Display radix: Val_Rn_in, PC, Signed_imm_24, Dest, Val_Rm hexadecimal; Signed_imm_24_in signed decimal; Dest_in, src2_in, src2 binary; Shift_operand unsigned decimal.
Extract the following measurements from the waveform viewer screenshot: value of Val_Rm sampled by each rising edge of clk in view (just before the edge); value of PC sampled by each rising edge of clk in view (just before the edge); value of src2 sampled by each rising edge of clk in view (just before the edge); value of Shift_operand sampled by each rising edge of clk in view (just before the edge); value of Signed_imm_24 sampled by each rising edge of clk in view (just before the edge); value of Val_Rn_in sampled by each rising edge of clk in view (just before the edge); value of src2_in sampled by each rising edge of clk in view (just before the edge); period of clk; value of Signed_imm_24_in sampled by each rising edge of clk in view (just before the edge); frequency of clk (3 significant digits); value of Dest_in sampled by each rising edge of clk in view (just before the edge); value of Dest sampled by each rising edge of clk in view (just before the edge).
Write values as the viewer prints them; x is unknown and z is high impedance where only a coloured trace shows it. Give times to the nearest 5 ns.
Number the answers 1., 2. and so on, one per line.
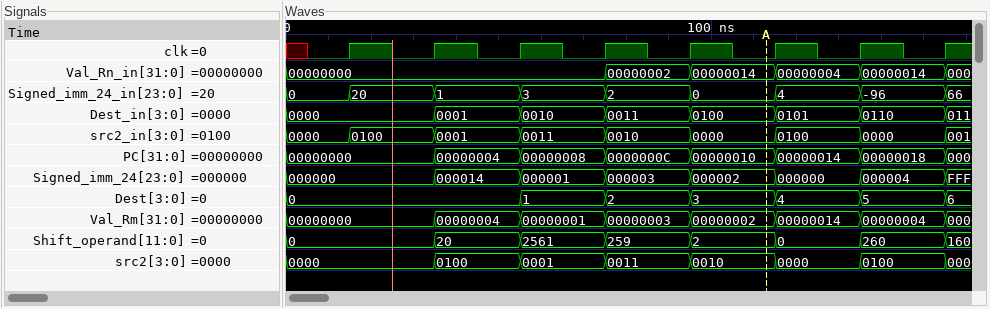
1. 00000000, 00000000, 00000004, 00000001, 00000003, 00000002, 00000014, 00000004
2. 00000000, 00000000, 00000004, 00000008, 0000000C, 00000010, 00000014, 00000018
3. 0000, 0000, 0100, 0001, 0011, 0010, 0000, 0100
4. 0, 0, 20, 2561, 259, 2, 0, 260
5. 000000, 000000, 000014, 000001, 000003, 000002, 000000, 000004
6. 00000000, 00000000, 00000000, 00000000, 00000002, 00000014, 00000004, 00000014
7. 0000, 0100, 0001, 0011, 0010, 0000, 0100, 0000
8. 20 ns
9. 0, 20, 1, 3, 2, 0, 4, -96
10. 50.0 MHz
11. 0000, 0000, 0001, 0010, 0011, 0100, 0101, 0110
12. 0, 0, 0, 1, 2, 3, 4, 5
